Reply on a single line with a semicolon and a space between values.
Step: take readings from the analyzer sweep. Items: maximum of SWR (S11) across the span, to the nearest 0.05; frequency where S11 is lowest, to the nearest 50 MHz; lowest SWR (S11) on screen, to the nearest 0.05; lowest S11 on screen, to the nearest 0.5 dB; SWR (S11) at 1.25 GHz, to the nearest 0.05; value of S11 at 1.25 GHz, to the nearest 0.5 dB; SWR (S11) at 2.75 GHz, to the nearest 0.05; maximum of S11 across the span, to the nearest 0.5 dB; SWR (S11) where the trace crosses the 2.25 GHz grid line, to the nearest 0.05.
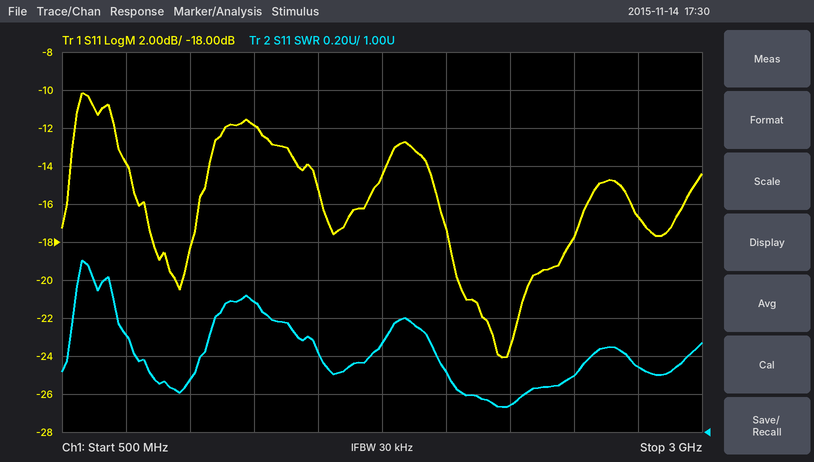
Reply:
1.90; 2.20 GHz; 1.15; -24.0 dB; 1.70; -12.0 dB; 1.35; -10.0 dB; 1.15
